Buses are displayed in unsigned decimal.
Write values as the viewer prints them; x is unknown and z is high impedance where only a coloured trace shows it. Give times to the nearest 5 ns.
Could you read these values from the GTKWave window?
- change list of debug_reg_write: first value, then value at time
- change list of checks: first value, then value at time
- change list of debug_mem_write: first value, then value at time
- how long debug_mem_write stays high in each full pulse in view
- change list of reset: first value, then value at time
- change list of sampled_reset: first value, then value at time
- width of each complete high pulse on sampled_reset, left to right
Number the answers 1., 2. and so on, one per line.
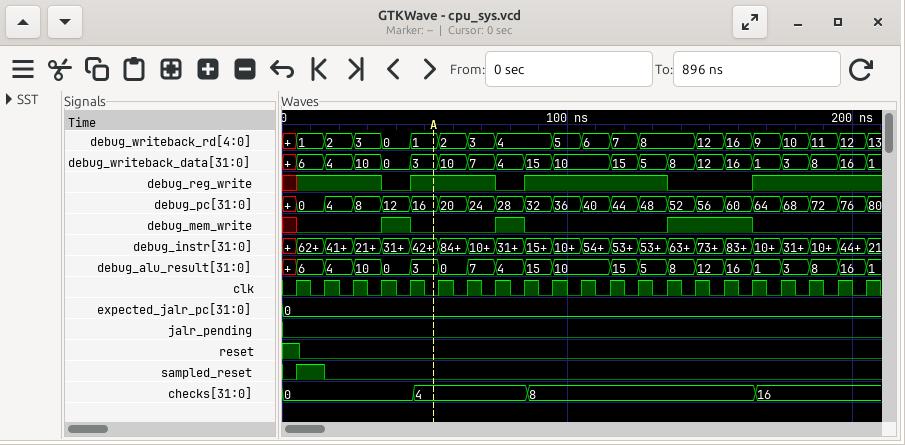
1. x, 1 at 5 ns, 0 at 35 ns, 1 at 45 ns, 0 at 75 ns, 1 at 85 ns, 0 at 135 ns, 1 at 165 ns
2. 0, 4 at 45 ns, 8 at 85 ns, 16 at 165 ns
3. x, 0 at 5 ns, 1 at 35 ns, 0 at 45 ns, 1 at 75 ns, 0 at 85 ns, 1 at 135 ns, 0 at 165 ns
4. 10 ns, 10 ns, 30 ns
5. 1, 0 at 5 ns
6. 0, 1 at 5 ns, 0 at 15 ns
7. 10 ns
